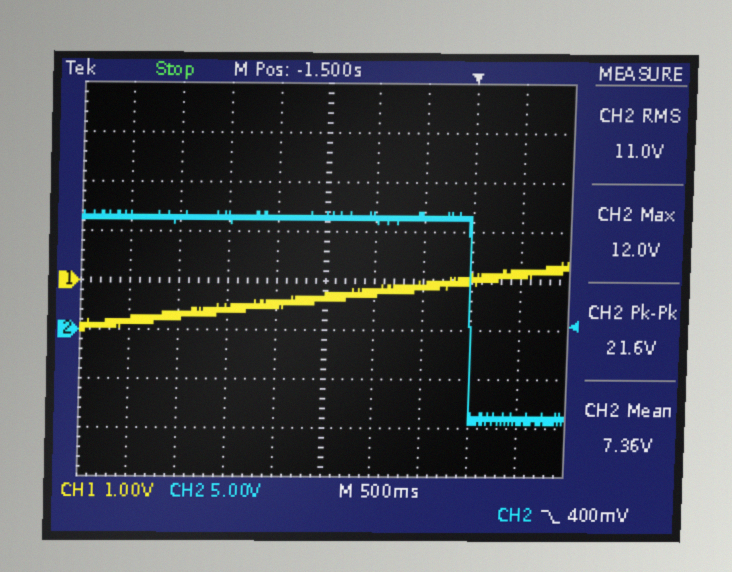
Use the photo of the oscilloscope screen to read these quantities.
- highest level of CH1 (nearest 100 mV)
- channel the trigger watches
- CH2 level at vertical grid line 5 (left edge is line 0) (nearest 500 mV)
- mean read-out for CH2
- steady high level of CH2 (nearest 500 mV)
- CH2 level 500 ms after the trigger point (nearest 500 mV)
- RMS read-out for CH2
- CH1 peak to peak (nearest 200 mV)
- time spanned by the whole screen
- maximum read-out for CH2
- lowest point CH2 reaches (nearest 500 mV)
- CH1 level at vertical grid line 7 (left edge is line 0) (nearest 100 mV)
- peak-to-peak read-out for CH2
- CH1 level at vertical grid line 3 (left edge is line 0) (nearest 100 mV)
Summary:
400 mV
CH2
11.5 V
7.36 V
11.5 V
-9.0 V
11.0 V
1.4 V
5 s
12.0 V
-9.5 V
-100 mV
21.6 V
-600 mV
